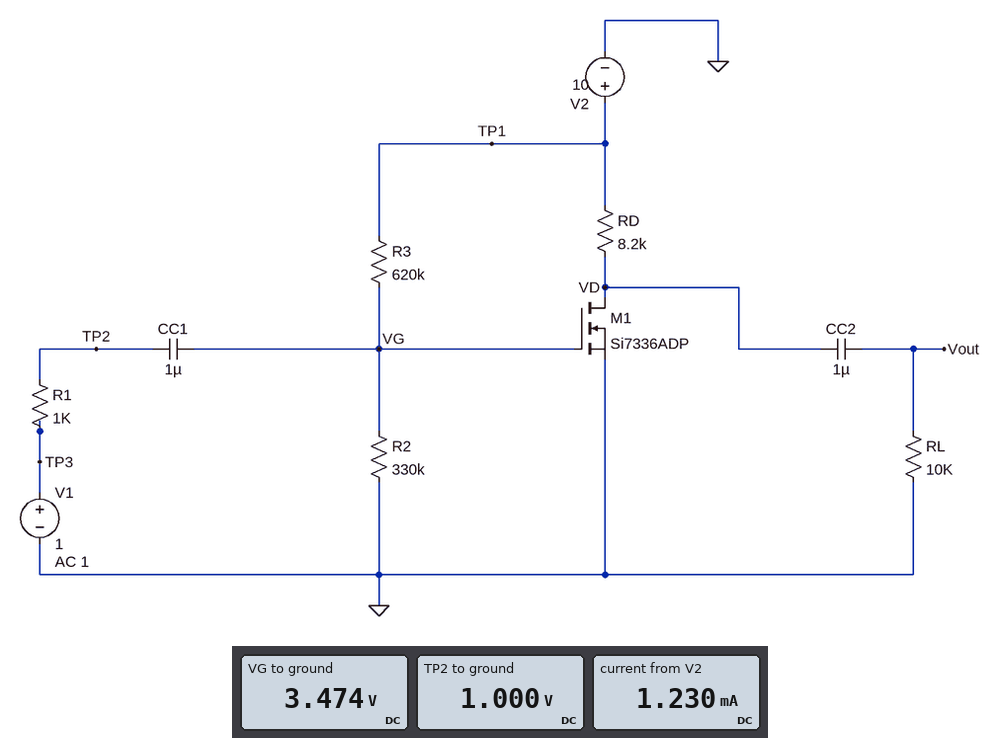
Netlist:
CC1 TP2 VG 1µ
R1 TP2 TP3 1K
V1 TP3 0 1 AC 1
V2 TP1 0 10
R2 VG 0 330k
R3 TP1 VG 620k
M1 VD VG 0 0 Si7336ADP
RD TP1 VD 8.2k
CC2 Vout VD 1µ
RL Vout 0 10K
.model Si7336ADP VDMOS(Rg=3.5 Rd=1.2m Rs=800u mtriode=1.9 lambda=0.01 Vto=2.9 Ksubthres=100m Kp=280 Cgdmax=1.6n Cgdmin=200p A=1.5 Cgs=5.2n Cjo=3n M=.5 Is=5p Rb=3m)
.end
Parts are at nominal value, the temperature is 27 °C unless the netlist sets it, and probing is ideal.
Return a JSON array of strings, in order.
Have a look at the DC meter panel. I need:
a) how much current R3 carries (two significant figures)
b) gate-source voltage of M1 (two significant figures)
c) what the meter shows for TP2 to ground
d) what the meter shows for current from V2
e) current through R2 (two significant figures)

["11 µA", "3.5 V", "1.000 V", "1.230 mA", "11 µA"]
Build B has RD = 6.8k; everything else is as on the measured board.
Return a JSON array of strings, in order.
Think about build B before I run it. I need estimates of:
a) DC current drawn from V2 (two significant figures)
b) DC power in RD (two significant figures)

["1.5 mA", "15 mW"]
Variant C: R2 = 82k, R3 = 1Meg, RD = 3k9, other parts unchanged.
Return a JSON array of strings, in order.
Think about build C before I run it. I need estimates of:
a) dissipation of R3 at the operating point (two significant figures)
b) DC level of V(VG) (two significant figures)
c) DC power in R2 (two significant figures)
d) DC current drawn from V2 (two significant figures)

["85 µW", "760 mV", "7.0 µW", "9.2 µA"]
